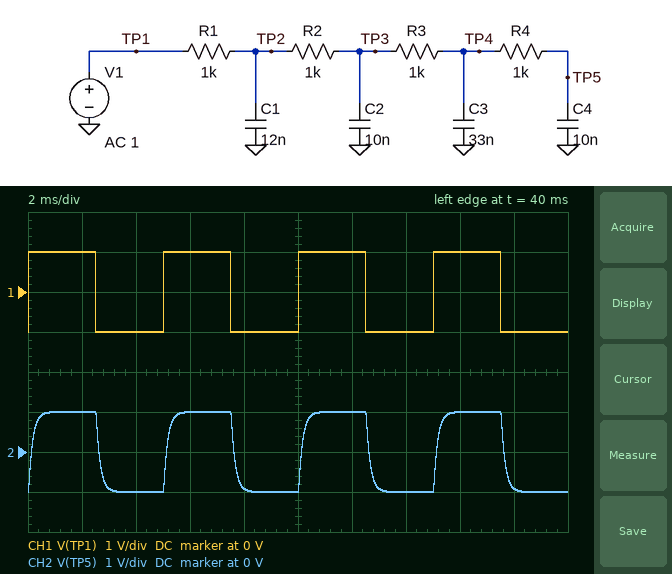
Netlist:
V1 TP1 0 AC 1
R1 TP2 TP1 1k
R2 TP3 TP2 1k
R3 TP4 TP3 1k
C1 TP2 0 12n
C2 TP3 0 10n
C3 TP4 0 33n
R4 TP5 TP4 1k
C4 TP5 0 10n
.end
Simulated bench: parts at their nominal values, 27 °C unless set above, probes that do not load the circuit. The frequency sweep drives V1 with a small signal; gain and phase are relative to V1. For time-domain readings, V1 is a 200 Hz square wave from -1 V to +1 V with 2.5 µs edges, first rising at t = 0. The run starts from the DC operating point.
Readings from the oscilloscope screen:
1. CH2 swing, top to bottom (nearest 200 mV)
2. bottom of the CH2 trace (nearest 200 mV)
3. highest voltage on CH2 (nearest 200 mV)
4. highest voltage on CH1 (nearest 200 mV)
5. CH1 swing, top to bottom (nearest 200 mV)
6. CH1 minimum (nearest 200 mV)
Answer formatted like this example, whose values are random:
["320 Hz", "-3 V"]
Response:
["2.0 V", "-1.0 V", "1.0 V", "1.0 V", "2.0 V", "-1.0 V"]
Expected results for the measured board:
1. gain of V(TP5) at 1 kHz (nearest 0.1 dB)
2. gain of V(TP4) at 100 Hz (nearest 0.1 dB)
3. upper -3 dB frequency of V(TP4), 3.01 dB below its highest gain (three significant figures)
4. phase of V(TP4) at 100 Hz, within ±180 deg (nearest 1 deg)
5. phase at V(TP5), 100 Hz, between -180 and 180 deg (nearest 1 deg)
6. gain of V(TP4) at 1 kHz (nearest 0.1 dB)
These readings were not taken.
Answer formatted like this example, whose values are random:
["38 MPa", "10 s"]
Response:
["-2.8 dB", "0 dB", "1.06 kHz", "-6 deg", "-6 deg", "-2.8 dB"]
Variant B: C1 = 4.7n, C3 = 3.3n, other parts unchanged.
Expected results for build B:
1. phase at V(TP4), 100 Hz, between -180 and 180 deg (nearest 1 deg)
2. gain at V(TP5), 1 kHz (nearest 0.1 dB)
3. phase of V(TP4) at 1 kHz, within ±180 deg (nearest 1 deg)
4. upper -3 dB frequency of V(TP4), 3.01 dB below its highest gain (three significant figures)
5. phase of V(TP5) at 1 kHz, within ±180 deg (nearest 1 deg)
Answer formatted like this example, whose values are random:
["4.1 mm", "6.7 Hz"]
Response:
["-2 deg", "-0.6 dB", "-22 deg", "2.56 kHz", "-26 deg"]
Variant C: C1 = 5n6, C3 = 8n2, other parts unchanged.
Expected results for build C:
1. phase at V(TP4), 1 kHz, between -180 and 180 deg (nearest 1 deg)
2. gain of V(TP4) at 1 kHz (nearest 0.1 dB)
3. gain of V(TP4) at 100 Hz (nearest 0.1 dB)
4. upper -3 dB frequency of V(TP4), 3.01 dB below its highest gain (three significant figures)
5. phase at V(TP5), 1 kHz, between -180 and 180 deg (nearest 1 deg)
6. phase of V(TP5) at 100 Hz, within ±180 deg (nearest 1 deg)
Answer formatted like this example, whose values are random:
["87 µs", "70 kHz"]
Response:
["-27 deg", "-0.9 dB", "0 dB", "2.09 kHz", "-31 deg", "-3 deg"]
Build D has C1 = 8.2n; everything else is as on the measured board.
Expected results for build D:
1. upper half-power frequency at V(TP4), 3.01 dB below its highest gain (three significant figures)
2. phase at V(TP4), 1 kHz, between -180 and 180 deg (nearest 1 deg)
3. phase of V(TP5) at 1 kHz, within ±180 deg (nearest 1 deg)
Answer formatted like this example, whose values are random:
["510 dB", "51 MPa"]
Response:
["1.07 kHz", "-46 deg", "-50 deg"]
